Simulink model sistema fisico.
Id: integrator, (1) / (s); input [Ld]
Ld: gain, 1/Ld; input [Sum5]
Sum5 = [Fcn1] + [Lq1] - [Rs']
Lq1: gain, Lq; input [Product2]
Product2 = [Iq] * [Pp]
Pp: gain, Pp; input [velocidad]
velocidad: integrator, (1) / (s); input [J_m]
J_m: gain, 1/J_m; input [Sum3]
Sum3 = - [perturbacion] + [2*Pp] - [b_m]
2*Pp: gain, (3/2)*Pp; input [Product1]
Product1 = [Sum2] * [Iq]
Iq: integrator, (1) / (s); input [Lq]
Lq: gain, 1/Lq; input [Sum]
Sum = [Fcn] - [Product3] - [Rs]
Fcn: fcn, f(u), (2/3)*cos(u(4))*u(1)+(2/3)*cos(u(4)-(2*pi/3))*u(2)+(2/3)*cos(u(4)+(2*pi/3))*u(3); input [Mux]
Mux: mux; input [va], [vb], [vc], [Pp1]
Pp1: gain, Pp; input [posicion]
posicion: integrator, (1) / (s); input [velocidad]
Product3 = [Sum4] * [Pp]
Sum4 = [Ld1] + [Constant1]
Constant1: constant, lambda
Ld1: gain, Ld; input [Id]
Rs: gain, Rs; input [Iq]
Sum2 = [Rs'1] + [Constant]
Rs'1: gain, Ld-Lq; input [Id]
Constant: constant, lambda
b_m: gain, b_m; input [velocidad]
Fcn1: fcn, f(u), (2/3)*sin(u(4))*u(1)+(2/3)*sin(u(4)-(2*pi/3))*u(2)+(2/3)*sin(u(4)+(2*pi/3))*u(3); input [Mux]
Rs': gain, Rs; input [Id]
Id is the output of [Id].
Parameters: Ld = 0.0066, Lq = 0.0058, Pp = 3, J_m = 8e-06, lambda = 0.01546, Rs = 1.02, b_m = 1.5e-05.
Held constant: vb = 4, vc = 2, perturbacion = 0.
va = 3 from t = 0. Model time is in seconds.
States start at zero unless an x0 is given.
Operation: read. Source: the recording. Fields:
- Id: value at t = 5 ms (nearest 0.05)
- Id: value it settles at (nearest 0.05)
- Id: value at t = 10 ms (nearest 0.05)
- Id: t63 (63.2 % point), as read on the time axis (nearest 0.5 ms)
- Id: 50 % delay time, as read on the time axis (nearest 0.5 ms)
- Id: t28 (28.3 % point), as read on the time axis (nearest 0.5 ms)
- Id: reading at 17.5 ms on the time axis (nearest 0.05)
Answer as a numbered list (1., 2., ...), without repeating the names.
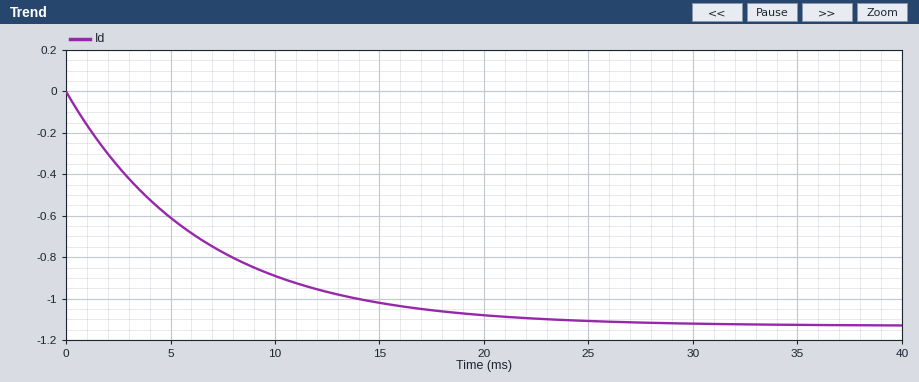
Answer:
1. -0.60
2. -1.15
3. -0.90
4. 6.5 ms
5. 4.5 ms
6. 2.0 ms
7. -1.05
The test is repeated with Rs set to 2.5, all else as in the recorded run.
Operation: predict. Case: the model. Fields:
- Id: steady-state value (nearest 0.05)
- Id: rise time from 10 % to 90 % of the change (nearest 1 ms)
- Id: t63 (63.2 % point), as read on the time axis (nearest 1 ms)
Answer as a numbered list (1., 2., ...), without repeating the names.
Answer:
1. -0.45
2. 6 ms
3. 3 ms
